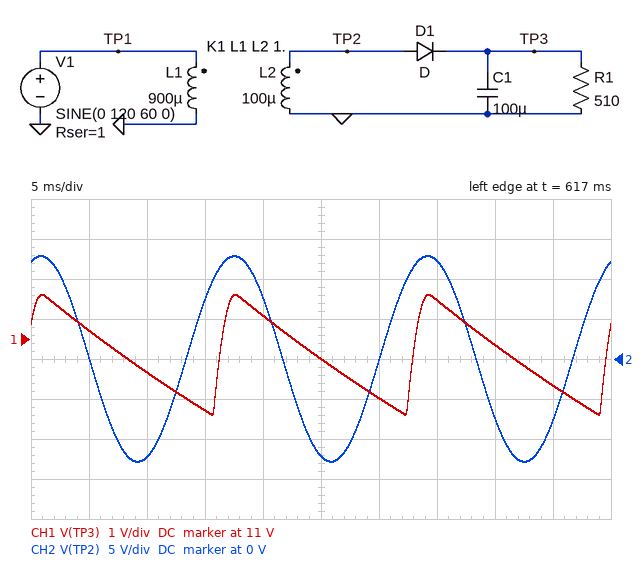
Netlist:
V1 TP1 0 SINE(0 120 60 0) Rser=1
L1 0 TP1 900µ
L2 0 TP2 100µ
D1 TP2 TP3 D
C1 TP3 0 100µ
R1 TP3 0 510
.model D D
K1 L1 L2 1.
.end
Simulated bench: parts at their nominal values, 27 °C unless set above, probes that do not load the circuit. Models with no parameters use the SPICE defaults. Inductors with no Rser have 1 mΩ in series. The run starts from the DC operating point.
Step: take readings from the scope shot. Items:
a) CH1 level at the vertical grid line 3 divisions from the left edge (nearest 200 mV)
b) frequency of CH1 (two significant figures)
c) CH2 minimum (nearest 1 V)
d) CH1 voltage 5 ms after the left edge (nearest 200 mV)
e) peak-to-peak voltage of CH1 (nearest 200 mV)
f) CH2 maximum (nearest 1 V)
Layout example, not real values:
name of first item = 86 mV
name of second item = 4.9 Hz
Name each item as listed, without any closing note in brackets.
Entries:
CH1 level at the vertical grid line 3 divisions from the left edge = 9.2 V
frequency of CH1 = 60 Hz
CH2 minimum = -13 V
CH1 voltage 5 ms after the left edge = 11.2 V
peak-to-peak voltage of CH1 = 3.0 V
CH2 maximum = 13 V
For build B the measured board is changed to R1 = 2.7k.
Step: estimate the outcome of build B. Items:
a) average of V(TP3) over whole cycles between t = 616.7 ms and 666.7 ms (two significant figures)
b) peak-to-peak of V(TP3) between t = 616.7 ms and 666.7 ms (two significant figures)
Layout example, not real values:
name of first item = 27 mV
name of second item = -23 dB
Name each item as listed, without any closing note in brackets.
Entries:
average of V(TP3) over whole cycles between t = 616.7 ms and 666.7 ms = 12 V
peak-to-peak of V(TP3) between t = 616.7 ms and 666.7 ms = 680 mV
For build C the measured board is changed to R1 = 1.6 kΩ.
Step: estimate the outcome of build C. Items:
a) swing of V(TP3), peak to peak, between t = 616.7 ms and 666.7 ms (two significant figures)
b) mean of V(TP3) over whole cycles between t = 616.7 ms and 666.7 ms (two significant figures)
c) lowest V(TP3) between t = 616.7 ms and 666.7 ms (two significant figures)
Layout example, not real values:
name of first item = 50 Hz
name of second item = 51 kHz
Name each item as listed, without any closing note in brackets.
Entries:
swing of V(TP3), peak to peak, between t = 616.7 ms and 666.7 ms = 1.1 V
mean of V(TP3) over whole cycles between t = 616.7 ms and 666.7 ms = 12 V
lowest V(TP3) between t = 616.7 ms and 666.7 ms = 11 V
